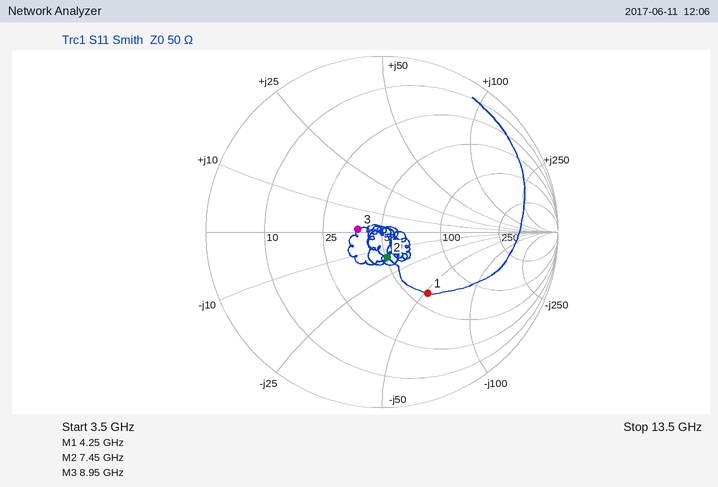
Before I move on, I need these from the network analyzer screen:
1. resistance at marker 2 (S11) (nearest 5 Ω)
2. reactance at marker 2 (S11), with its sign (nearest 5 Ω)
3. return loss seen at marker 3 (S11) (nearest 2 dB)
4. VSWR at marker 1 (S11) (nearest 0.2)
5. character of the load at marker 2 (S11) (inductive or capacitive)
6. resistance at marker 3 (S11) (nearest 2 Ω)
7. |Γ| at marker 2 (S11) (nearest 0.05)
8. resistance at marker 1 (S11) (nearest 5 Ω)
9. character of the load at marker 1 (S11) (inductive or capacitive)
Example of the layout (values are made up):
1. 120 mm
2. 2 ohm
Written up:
1. 50 Ω
2. -15 Ω
3. 18 dB
4. 2.6
5. capacitive
6. 38 Ω
7. 0.15
8. 60 Ω
9. capacitive
